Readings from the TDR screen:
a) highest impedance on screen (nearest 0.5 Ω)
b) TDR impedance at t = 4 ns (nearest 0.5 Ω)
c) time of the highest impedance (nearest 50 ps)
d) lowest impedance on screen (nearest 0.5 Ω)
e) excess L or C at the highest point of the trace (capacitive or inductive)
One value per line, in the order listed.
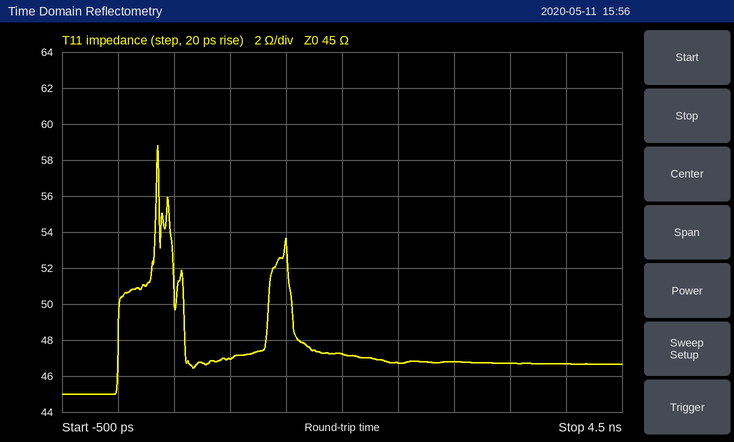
59.0 Ω
46.5 Ω
350 ps
45.0 Ω
inductive
